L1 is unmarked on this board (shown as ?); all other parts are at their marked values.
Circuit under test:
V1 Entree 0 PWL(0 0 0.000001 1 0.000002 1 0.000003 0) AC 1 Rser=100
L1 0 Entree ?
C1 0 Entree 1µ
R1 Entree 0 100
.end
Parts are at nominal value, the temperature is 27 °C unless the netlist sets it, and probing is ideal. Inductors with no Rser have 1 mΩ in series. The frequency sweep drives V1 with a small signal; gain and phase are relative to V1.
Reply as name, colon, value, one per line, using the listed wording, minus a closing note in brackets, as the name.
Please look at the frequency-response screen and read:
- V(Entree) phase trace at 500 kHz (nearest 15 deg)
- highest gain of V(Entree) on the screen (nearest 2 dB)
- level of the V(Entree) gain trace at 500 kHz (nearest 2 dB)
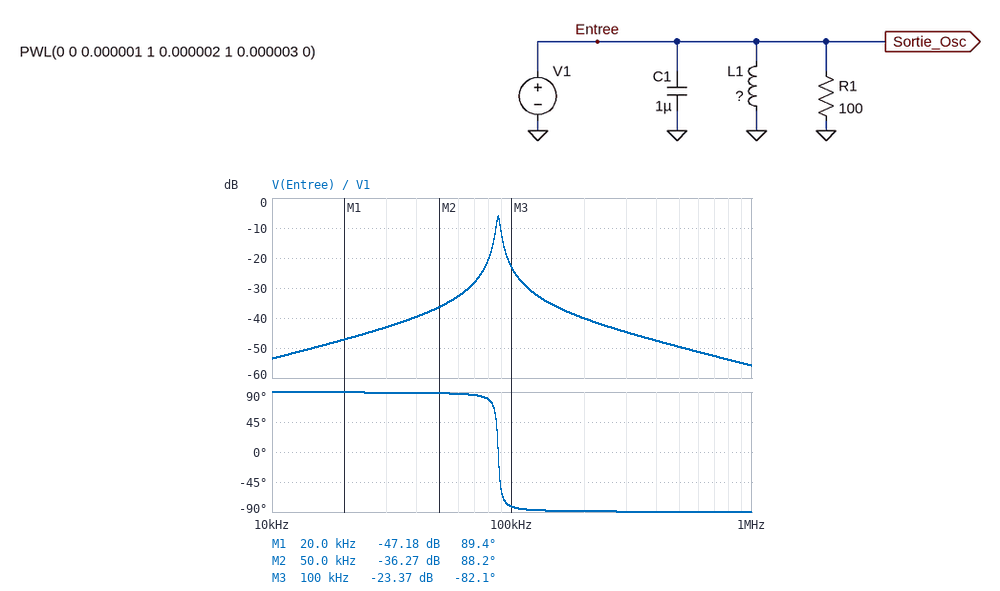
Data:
V(Entree) phase trace at 500 kHz: -90 deg
highest gain of V(Entree) on the screen: -6 dB
level of the V(Entree) gain trace at 500 kHz: -50 dB
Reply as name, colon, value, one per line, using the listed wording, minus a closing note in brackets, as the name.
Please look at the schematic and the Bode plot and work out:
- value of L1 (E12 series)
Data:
value of L1: 3.3 µH
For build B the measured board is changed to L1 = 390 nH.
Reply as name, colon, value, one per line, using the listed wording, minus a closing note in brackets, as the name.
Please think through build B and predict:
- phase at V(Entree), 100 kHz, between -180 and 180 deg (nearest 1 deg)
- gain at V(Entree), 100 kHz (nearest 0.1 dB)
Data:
phase at V(Entree), 100 kHz, between -180 and 180 deg: 89 deg
gain at V(Entree), 100 kHz: -50.8 dB
